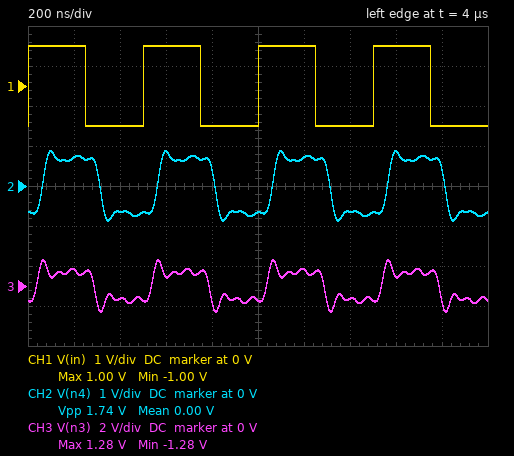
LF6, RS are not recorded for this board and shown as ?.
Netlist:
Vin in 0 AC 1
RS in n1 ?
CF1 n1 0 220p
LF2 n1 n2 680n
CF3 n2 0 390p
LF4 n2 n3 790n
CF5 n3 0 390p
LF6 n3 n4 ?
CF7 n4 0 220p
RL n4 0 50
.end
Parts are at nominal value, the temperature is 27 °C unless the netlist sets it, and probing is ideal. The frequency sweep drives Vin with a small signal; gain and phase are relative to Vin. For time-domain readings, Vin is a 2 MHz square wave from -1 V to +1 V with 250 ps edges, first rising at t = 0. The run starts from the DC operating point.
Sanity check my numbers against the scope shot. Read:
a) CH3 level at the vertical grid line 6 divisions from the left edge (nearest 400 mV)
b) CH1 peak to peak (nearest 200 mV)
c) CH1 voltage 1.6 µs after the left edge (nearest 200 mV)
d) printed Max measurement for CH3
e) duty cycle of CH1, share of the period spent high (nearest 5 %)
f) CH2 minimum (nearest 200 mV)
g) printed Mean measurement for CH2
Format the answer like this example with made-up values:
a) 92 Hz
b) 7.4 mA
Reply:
a) 800 mV
b) 2.0 V
c) 1.0 V
d) 1.28 V
e) 50 %
f) -800 mV
g) 0.00 V
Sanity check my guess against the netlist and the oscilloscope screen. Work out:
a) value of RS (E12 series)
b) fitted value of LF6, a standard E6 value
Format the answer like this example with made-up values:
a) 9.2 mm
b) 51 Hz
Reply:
a) 22 Ω
b) 1.5 µH
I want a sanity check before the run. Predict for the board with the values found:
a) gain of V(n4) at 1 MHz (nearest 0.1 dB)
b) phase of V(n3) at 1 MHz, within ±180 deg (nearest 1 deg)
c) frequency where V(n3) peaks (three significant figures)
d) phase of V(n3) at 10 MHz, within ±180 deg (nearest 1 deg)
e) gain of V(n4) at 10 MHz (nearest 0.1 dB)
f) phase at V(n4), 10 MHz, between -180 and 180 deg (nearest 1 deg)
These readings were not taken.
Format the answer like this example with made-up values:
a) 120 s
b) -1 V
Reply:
a) -3.2 dB
b) -11 deg
c) 15.5 MHz
d) -142 deg
e) -4.2 dB
f) 119 deg
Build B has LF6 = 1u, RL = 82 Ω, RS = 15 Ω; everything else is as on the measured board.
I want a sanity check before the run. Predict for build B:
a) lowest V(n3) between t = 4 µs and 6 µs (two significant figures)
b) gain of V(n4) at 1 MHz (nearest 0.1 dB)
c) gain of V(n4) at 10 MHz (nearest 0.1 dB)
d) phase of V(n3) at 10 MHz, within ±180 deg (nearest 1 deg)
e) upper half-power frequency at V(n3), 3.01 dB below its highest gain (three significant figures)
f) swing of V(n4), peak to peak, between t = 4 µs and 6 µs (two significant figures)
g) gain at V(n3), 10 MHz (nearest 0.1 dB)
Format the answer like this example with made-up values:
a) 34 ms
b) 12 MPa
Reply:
a) -1.2 V
b) -1.3 dB
c) 0 dB
d) -127 deg
e) 16.7 MHz
f) 2.9 V
g) -2.2 dB
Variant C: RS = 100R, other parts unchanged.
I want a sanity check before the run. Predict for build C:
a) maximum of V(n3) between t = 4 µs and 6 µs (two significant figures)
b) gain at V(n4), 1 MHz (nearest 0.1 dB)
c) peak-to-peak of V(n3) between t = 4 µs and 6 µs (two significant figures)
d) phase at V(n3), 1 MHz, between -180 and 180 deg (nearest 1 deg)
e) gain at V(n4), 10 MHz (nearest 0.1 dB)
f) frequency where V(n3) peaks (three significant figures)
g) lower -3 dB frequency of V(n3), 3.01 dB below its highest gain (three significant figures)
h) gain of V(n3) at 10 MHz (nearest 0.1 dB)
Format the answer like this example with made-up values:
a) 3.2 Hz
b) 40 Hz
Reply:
a) 610 mV
b) -9.5 dB
c) 1.2 V
d) -11 deg
e) -11.1 dB
f) 12.1 MHz
g) 10.2 MHz
h) -5.5 dB
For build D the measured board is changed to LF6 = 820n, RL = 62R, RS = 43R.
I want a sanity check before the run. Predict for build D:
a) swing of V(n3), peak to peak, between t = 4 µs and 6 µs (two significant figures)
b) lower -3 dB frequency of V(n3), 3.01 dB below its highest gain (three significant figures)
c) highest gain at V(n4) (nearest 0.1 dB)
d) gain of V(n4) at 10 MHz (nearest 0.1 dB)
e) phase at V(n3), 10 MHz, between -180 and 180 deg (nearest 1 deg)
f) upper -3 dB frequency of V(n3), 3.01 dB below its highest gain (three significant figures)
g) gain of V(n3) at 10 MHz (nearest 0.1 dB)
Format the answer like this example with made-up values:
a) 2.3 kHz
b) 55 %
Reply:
a) 1.5 V
b) 13.4 MHz
c) -4.4 dB
d) -4.5 dB
e) -130 deg
f) 17.6 MHz
g) -5.6 dB
